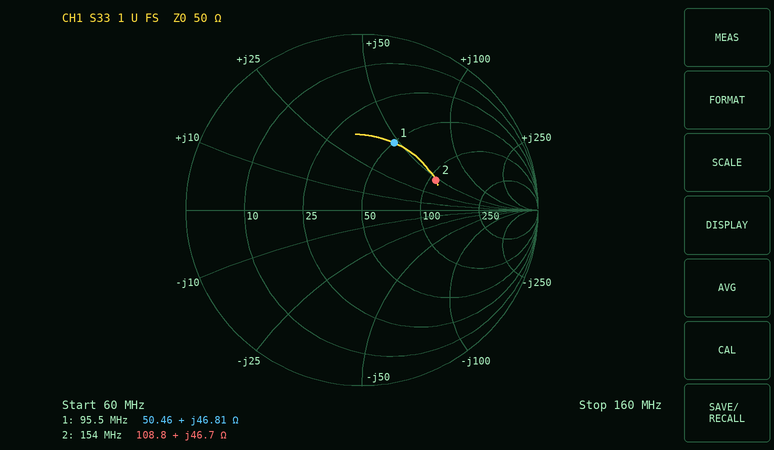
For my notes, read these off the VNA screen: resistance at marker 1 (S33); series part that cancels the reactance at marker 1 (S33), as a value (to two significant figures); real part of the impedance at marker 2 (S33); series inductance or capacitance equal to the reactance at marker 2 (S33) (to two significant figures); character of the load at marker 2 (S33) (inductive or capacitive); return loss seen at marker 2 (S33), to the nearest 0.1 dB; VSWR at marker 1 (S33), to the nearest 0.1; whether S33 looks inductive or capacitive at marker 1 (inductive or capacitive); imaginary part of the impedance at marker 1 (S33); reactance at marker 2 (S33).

50.46 Ω
36 pF
108.8 Ω
48 nH
inductive
6.9 dB
2.5
inductive
+46.81 Ω
+46.7 Ω
